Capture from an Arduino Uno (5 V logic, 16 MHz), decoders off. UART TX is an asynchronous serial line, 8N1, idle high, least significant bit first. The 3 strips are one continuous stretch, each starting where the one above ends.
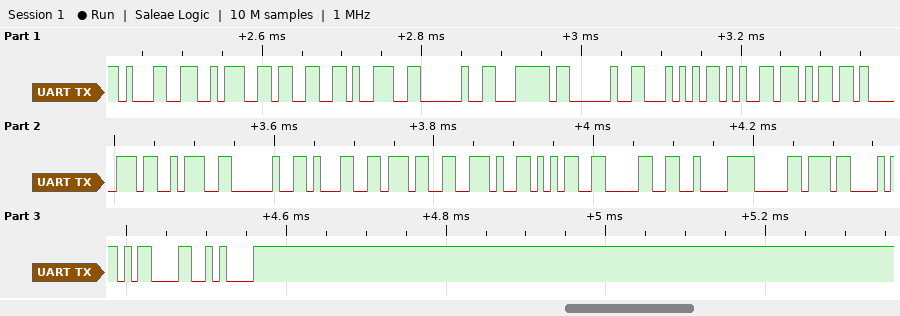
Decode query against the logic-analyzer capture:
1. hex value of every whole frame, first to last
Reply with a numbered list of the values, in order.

1. 0x31 0x3A 0x33 0x39 0x20 0x7C 0x20 0x54 0x65 0x6D 0x70 0x3A 0x20 0x31 0x37 0x2E 0x35 0x30 0xC2 0xB0 0x43 0x0D 0x0A
